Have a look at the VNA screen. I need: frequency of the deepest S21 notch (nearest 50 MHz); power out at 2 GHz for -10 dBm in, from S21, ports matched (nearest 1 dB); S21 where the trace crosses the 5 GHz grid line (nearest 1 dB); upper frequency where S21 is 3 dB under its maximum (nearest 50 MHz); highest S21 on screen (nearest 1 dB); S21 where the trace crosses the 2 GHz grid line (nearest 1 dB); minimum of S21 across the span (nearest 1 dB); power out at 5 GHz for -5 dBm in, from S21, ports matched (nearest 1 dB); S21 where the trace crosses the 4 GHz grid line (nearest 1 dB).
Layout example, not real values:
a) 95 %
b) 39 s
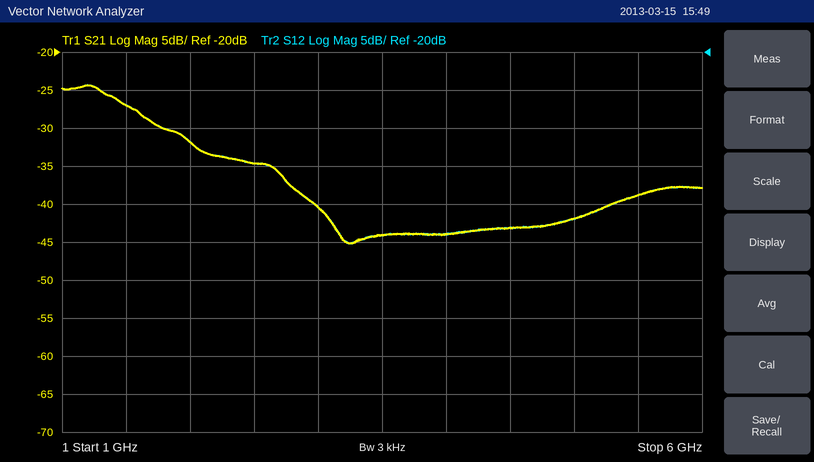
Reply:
a) 3.25 GHz
b) -42 dBm
c) -42 dB
d) 1.55 GHz
e) -24 dB
f) -32 dB
g) -45 dB
h) -47 dBm
i) -44 dB
